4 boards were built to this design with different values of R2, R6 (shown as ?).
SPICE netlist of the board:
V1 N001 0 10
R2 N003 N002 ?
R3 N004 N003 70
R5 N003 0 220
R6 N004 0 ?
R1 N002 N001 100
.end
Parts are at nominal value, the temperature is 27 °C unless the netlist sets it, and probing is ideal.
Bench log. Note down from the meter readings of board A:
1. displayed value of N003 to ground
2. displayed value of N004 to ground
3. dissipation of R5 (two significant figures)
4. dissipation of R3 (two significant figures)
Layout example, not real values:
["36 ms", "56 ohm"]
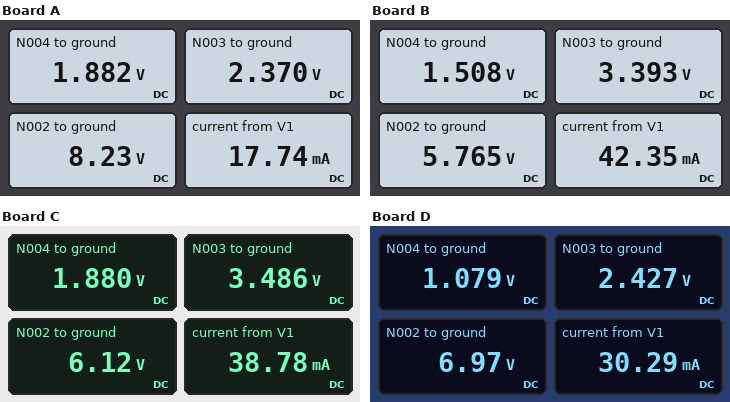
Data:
["2.370 V", "1.882 V", "26 mW", "3.4 mW"]
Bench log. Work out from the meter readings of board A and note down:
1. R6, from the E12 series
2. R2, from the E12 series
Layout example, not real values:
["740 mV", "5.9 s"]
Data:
["270 Ω", "330 Ω"]
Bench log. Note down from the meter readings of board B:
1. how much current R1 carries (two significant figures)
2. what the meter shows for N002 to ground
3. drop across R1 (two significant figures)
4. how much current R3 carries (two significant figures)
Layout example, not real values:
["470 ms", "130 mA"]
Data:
["42 mA", "5.765 V", "4.2 V", "27 mA"]
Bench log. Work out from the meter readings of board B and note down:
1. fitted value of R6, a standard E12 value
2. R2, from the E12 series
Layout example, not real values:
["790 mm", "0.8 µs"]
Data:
["56 Ω", "56 Ω"]
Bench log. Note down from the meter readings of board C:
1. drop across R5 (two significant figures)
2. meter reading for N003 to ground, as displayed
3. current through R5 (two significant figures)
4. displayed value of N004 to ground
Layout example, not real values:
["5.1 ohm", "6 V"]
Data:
["3.5 V", "3.486 V", "16 mA", "1.880 V"]
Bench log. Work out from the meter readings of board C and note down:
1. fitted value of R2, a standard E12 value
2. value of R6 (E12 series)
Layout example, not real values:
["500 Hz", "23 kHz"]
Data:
["68 Ω", "82 Ω"]
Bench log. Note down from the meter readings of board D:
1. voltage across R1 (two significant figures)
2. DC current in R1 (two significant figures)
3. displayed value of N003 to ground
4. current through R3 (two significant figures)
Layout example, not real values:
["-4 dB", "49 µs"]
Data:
["3.0 V", "30 mA", "2.427 V", "19 mA"]
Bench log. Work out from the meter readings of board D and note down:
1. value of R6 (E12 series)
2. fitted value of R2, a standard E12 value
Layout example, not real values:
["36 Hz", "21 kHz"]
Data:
["56 Ω", "150 Ω"]
